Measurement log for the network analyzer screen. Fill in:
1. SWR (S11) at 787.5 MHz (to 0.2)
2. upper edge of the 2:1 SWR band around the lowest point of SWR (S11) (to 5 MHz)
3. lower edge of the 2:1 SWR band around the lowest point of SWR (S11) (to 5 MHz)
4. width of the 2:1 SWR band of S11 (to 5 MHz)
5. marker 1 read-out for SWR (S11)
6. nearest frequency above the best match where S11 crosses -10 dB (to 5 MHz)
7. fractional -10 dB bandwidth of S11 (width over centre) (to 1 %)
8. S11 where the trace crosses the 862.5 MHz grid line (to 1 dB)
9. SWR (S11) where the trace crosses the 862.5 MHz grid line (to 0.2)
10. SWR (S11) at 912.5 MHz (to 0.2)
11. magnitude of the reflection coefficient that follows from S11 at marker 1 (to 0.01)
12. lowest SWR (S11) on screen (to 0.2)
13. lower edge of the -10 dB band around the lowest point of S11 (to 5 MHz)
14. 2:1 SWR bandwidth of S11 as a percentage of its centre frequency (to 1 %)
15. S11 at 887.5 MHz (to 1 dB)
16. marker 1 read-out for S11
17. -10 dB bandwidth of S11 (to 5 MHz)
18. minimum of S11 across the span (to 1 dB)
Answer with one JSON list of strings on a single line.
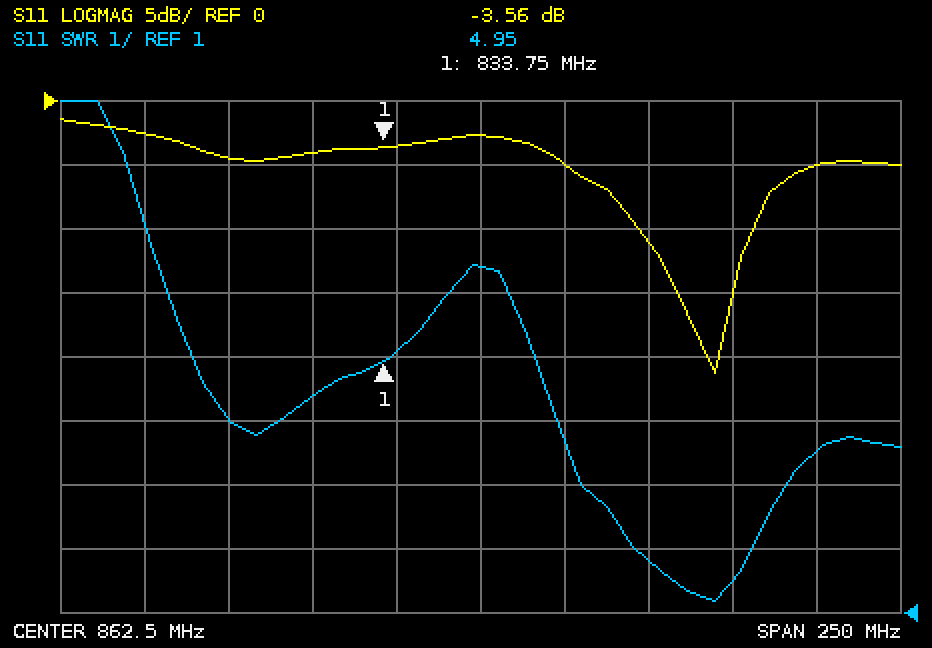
["4.0", "945 MHz", "910 MHz", "35 MHz", "4.95", "945 MHz", "4 %", "-3 dB", "6.4", "1.8", "0.66", "1.2", "910 MHz", "4 %", "-5 dB", "-3.56 dB", "35 MHz", "-21 dB"]
